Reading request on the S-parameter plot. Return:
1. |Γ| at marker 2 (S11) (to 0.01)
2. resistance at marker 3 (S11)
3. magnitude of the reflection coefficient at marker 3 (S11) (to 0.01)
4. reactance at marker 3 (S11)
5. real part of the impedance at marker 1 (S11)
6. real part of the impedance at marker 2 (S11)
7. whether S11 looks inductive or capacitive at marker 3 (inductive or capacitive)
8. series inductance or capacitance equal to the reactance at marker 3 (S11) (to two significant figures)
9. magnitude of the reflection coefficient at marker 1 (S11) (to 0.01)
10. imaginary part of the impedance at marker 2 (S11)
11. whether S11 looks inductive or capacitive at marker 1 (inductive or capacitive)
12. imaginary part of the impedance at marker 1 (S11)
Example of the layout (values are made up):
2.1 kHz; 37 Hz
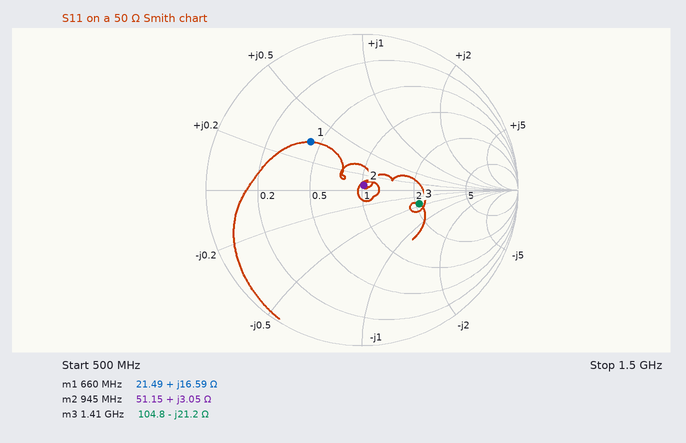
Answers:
0.03; 104.8 Ω; 0.38; -21.2 Ω; 21.49 Ω; 51.15 Ω; capacitive; 5.3 pF; 0.45; +3.05 Ω; inductive; +16.59 Ω
